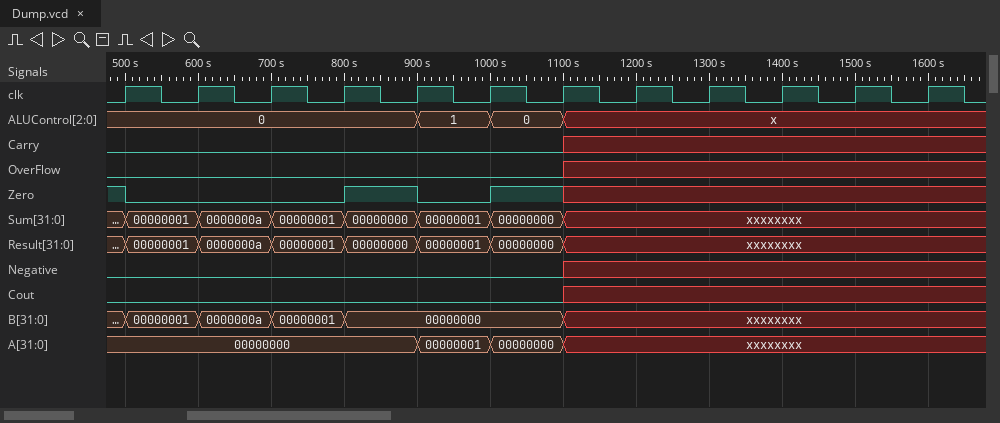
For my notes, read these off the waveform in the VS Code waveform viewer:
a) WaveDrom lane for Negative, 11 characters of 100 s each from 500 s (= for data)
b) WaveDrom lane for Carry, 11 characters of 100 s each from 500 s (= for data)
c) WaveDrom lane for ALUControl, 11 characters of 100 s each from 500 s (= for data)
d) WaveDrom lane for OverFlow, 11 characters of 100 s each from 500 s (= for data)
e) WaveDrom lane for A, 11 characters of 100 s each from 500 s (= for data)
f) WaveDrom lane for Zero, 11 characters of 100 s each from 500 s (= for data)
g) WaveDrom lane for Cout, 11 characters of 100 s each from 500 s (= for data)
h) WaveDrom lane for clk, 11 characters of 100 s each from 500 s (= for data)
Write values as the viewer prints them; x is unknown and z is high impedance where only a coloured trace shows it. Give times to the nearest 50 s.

{name: 'Negative', wave: '0.....x....'}
{name: 'Carry', wave: '0.....x....'}
{name: 'ALUControl', wave: '=...==x....', data: '0 1 0'}
{name: 'OverFlow', wave: '0.....x....'}
{name: 'A', wave: '=...==x....', data: '00000000 00000001 00000000'}
{name: 'Zero', wave: '0..101x....'}
{name: 'Cout', wave: '0.....x....'}
{name: 'clk', wave: 'p..........'}
